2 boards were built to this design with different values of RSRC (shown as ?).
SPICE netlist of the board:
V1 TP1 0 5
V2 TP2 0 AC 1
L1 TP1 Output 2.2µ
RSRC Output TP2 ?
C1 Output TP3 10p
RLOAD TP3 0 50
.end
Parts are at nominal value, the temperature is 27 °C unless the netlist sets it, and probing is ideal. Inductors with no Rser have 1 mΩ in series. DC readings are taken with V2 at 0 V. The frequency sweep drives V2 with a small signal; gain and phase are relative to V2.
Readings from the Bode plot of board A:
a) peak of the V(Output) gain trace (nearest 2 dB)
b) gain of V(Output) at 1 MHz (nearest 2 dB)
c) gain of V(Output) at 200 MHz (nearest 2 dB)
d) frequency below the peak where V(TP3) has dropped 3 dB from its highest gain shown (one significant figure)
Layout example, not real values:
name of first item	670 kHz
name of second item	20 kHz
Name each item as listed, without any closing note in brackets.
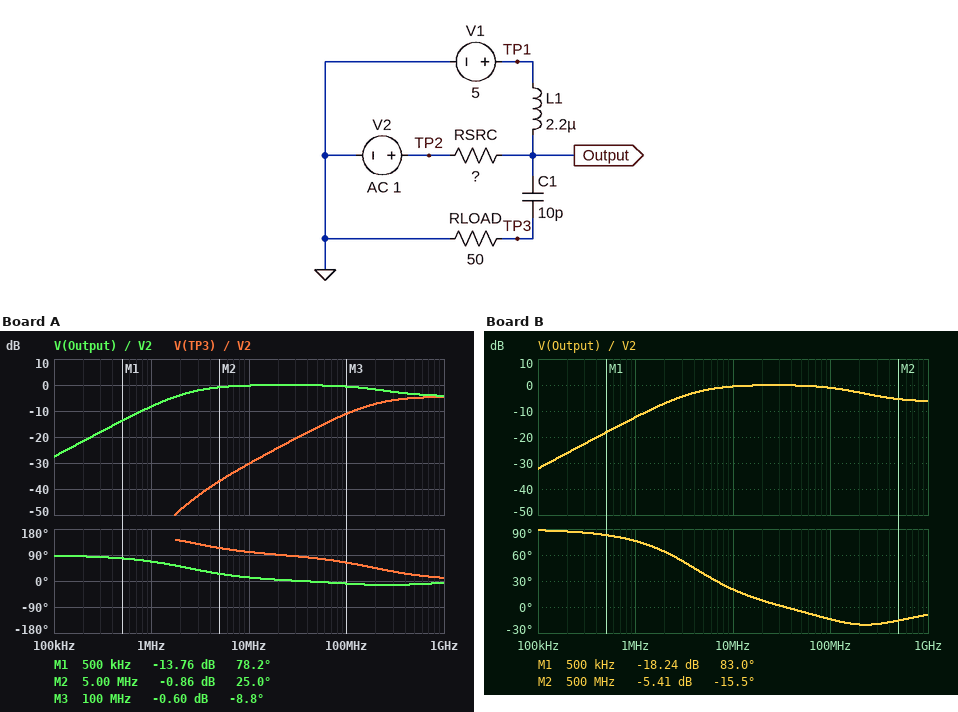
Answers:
peak of the V(Output) gain trace	0 dB
gain of V(Output) at 1 MHz	-8 dB
gain of V(Output) at 200 MHz	-2 dB
frequency below the peak where V(TP3) has dropped 3 dB from its highest gain shown	200 MHz
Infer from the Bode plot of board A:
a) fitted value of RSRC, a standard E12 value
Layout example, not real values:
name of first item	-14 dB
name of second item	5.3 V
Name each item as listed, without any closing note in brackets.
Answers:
fitted value of RSRC, a standard E12 value	33 Ω
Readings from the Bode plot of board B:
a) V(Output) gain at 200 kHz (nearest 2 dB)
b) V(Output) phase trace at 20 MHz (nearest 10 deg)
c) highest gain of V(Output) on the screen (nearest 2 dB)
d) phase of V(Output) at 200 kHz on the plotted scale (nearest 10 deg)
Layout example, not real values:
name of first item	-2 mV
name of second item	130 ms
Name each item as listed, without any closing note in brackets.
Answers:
V(Output) gain at 200 kHz	-26 dB
V(Output) phase trace at 20 MHz	10 deg
highest gain of V(Output) on the screen	0 dB
phase of V(Output) at 200 kHz on the plotted scale	90 deg
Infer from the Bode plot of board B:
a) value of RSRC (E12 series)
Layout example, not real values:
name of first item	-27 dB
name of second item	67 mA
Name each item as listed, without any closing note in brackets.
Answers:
value of RSRC	56 Ω
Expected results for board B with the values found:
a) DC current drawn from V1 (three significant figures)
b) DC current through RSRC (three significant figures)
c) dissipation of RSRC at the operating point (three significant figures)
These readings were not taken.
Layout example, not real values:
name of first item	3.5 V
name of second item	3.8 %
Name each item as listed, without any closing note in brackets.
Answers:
DC current drawn from V1	89.3 mA
DC current through RSRC	89.3 mA
dissipation of RSRC at the operating point	446 mW
